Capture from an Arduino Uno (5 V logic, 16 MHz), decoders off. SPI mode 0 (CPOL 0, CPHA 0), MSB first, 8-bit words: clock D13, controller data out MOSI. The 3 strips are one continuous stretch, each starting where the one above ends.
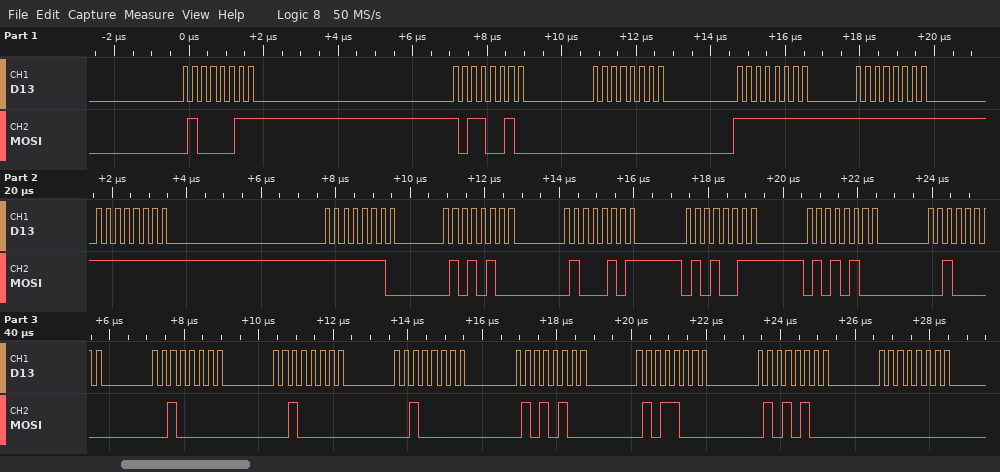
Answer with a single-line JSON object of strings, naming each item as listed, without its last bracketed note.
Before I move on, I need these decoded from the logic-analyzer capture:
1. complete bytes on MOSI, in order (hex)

{"complete bytes on MOSI, in order": "0x43 0xB2 0x00 0xFF 0xFF 0xFF 0xFE 0x54 0x45 0x53 0x54 0x20 0x20 0x20 0x20 0x54 0x58 0x54 0x00"}
